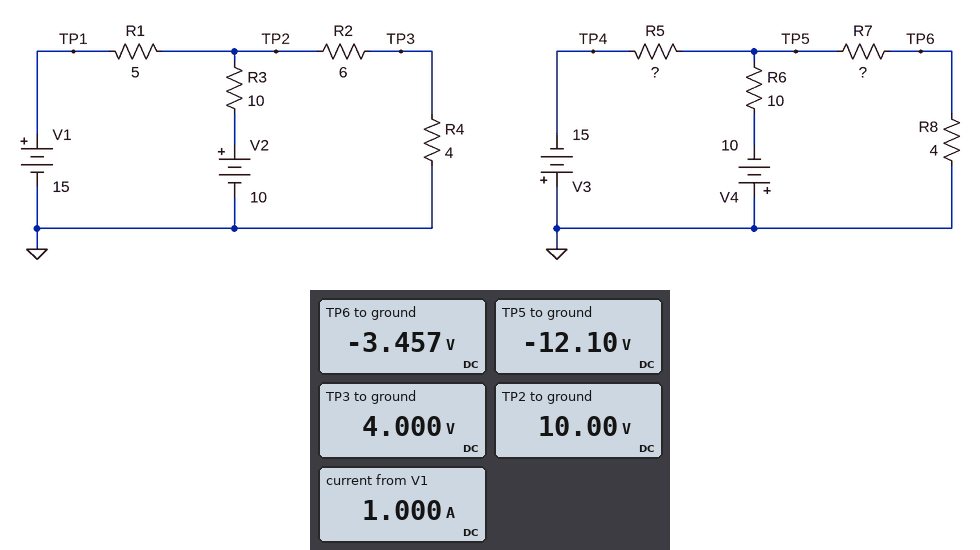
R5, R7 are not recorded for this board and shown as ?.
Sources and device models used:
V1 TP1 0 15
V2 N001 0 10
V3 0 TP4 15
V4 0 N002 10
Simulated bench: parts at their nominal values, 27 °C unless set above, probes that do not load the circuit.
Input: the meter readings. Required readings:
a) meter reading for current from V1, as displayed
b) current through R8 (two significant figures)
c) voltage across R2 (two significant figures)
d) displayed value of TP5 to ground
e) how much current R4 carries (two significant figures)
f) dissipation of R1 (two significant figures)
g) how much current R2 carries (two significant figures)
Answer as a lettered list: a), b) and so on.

a) 1.000 A
b) 860 mA
c) 6.0 V
d) -12.10 V
e) 1.0 A
f) 5.0 W
g) 1.0 A
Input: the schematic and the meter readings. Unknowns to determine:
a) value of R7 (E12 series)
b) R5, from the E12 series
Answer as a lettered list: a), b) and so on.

a) 10 Ω
b) 2.7 Ω
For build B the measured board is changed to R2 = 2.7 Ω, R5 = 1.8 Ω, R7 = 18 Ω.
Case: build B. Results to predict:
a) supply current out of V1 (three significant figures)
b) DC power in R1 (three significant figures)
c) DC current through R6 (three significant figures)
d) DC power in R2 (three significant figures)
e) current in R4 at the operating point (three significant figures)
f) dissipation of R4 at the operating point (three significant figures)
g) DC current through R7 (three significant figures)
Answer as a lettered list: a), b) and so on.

a) 1.22 A
b) 7.43 W
c) 331 mA
d) 4.77 W
e) 1.33 A
f) 7.06 W
g) 605 mA
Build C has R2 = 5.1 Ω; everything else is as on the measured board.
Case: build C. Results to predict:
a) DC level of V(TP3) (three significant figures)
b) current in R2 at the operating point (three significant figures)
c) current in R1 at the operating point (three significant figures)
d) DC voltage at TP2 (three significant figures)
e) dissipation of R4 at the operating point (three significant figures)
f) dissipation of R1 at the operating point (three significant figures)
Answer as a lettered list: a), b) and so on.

a) 4.29 V
b) 1.07 A
c) 1.05 A
d) 9.76 V
e) 4.60 W
f) 5.49 W
